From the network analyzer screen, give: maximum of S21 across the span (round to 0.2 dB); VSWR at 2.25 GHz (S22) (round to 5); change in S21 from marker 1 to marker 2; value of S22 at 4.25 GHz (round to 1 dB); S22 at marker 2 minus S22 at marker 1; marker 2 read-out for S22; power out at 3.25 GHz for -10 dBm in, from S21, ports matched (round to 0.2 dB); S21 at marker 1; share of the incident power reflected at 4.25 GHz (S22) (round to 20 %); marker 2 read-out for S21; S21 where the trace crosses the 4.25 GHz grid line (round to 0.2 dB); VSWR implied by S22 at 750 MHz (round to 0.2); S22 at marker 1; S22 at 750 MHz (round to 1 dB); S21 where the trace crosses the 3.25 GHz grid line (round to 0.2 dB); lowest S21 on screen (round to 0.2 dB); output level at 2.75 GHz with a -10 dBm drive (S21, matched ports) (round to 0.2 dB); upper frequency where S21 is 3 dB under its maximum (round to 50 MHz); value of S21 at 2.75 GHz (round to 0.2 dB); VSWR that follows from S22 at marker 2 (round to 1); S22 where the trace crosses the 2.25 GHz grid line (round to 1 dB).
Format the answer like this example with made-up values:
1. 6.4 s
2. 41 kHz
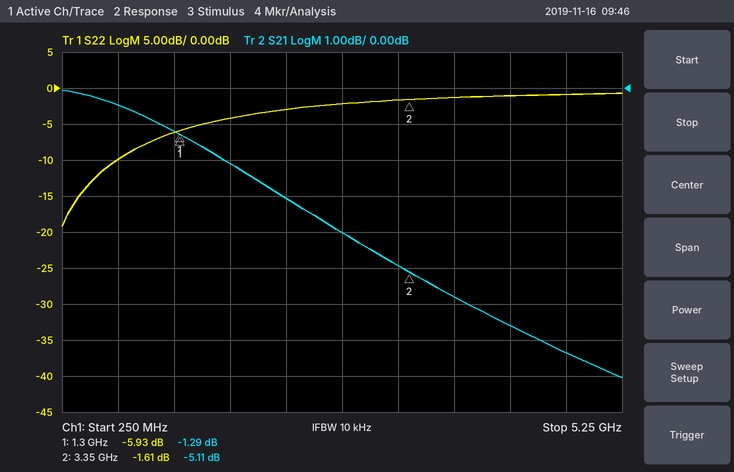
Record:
1. 0.0 dB
2. 5
3. -3.82 dB
4. -1 dB
5. 4.32 dB
6. -1.61 dB
7. -15.0 dBm
8. -1.29 dB
9. 80 %
10. -5.11 dB
11. -6.6 dB
12. 2.0
13. -5.93 dB
14. -10 dB
15. -5.0 dB
16. -8.0 dB
17. -14.0 dBm
18. 2.25 GHz
19. -4.0 dB
20. 11
21. -3 dB
